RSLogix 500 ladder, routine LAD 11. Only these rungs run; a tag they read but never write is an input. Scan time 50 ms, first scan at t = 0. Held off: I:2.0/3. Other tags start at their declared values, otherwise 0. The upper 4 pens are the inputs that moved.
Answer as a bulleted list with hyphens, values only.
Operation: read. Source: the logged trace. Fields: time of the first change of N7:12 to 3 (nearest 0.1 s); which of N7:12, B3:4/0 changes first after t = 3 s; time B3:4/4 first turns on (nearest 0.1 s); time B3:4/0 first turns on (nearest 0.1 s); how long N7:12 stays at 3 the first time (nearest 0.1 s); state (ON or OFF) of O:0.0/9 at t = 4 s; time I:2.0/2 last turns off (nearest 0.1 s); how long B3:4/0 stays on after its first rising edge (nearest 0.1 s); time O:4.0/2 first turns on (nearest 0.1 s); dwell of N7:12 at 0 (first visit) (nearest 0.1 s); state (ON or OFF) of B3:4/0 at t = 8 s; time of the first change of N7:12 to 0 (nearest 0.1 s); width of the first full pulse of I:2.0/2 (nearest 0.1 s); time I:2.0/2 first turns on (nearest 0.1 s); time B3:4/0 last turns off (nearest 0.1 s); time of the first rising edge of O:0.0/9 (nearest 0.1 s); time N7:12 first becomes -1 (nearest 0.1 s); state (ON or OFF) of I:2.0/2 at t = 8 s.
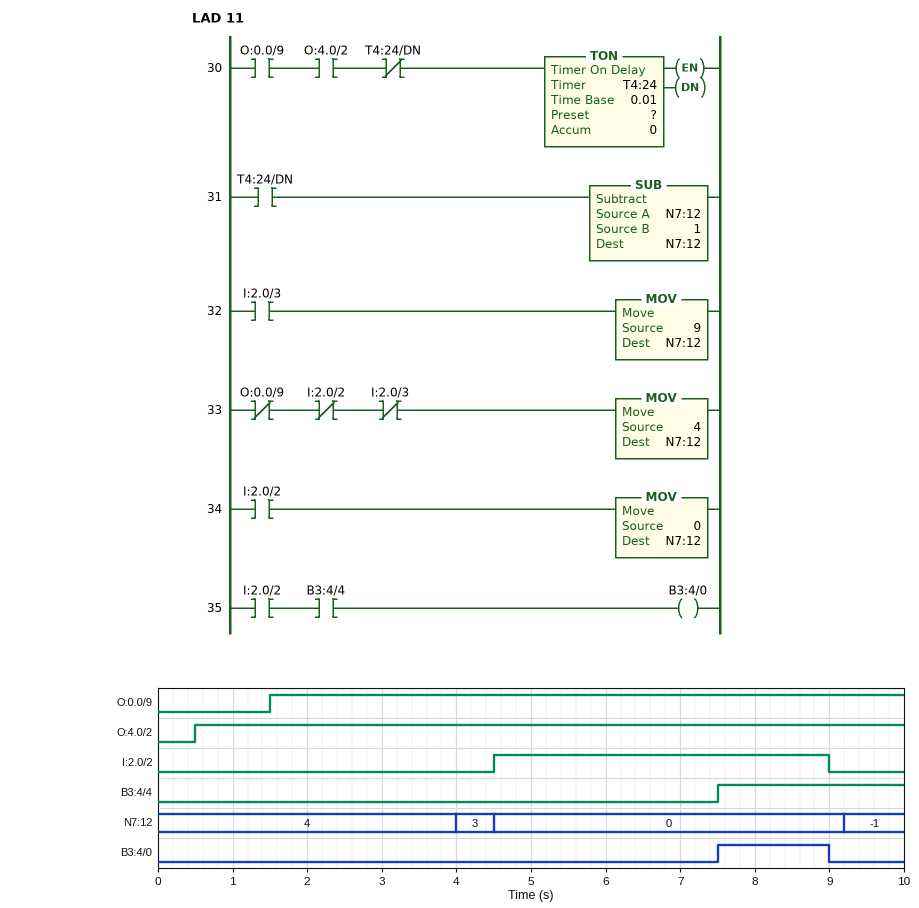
- 4.0 s
- N7:12
- 7.5 s
- 7.5 s
- 0.5 s
- ON
- 9.0 s
- 1.5 s
- 0.5 s
- 4.7 s
- ON
- 4.5 s
- 4.5 s
- 4.5 s
- 9.0 s
- 1.5 s
- 9.2 s
- ON
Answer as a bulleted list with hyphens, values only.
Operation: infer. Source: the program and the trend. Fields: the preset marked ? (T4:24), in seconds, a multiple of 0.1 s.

- 2.5 s
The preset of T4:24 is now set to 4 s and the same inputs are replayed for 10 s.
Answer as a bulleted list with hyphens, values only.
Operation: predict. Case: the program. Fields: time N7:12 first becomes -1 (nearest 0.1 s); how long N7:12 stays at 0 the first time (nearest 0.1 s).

- 9.6 s
- 5.1 s
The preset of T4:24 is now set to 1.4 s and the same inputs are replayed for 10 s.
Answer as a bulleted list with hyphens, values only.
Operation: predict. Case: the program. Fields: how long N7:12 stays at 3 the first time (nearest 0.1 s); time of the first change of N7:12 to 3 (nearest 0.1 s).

- 1.5 s
- 2.9 s
